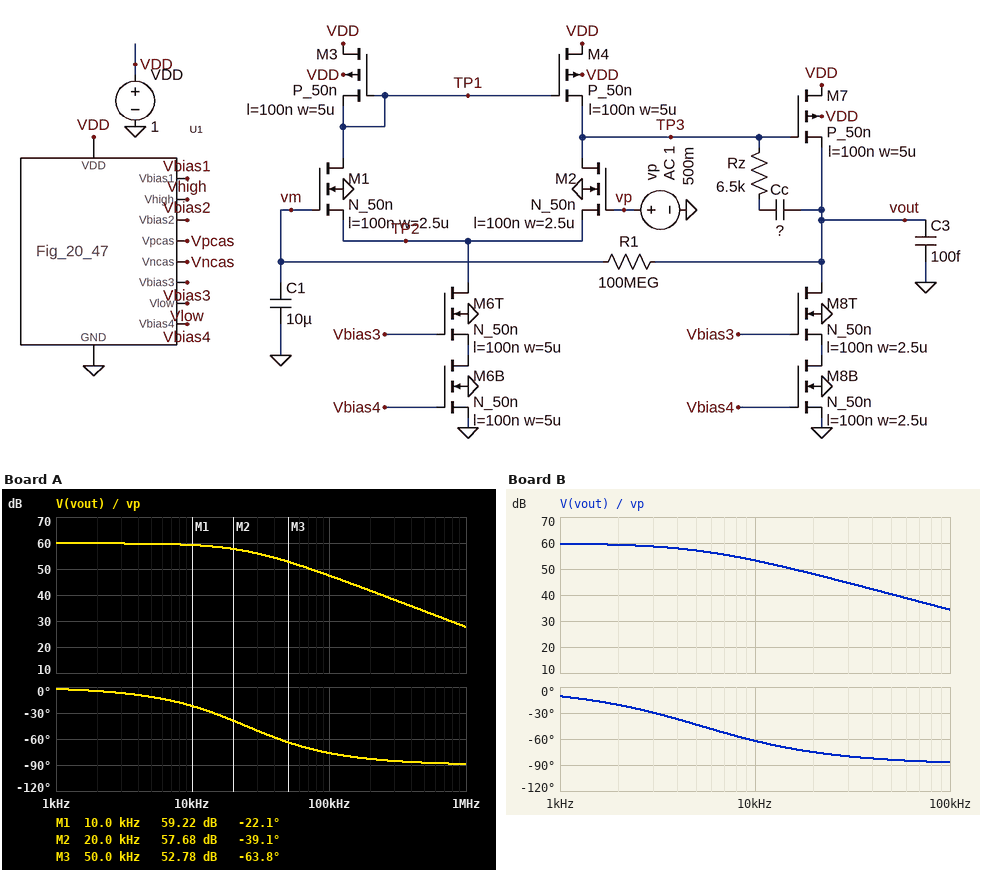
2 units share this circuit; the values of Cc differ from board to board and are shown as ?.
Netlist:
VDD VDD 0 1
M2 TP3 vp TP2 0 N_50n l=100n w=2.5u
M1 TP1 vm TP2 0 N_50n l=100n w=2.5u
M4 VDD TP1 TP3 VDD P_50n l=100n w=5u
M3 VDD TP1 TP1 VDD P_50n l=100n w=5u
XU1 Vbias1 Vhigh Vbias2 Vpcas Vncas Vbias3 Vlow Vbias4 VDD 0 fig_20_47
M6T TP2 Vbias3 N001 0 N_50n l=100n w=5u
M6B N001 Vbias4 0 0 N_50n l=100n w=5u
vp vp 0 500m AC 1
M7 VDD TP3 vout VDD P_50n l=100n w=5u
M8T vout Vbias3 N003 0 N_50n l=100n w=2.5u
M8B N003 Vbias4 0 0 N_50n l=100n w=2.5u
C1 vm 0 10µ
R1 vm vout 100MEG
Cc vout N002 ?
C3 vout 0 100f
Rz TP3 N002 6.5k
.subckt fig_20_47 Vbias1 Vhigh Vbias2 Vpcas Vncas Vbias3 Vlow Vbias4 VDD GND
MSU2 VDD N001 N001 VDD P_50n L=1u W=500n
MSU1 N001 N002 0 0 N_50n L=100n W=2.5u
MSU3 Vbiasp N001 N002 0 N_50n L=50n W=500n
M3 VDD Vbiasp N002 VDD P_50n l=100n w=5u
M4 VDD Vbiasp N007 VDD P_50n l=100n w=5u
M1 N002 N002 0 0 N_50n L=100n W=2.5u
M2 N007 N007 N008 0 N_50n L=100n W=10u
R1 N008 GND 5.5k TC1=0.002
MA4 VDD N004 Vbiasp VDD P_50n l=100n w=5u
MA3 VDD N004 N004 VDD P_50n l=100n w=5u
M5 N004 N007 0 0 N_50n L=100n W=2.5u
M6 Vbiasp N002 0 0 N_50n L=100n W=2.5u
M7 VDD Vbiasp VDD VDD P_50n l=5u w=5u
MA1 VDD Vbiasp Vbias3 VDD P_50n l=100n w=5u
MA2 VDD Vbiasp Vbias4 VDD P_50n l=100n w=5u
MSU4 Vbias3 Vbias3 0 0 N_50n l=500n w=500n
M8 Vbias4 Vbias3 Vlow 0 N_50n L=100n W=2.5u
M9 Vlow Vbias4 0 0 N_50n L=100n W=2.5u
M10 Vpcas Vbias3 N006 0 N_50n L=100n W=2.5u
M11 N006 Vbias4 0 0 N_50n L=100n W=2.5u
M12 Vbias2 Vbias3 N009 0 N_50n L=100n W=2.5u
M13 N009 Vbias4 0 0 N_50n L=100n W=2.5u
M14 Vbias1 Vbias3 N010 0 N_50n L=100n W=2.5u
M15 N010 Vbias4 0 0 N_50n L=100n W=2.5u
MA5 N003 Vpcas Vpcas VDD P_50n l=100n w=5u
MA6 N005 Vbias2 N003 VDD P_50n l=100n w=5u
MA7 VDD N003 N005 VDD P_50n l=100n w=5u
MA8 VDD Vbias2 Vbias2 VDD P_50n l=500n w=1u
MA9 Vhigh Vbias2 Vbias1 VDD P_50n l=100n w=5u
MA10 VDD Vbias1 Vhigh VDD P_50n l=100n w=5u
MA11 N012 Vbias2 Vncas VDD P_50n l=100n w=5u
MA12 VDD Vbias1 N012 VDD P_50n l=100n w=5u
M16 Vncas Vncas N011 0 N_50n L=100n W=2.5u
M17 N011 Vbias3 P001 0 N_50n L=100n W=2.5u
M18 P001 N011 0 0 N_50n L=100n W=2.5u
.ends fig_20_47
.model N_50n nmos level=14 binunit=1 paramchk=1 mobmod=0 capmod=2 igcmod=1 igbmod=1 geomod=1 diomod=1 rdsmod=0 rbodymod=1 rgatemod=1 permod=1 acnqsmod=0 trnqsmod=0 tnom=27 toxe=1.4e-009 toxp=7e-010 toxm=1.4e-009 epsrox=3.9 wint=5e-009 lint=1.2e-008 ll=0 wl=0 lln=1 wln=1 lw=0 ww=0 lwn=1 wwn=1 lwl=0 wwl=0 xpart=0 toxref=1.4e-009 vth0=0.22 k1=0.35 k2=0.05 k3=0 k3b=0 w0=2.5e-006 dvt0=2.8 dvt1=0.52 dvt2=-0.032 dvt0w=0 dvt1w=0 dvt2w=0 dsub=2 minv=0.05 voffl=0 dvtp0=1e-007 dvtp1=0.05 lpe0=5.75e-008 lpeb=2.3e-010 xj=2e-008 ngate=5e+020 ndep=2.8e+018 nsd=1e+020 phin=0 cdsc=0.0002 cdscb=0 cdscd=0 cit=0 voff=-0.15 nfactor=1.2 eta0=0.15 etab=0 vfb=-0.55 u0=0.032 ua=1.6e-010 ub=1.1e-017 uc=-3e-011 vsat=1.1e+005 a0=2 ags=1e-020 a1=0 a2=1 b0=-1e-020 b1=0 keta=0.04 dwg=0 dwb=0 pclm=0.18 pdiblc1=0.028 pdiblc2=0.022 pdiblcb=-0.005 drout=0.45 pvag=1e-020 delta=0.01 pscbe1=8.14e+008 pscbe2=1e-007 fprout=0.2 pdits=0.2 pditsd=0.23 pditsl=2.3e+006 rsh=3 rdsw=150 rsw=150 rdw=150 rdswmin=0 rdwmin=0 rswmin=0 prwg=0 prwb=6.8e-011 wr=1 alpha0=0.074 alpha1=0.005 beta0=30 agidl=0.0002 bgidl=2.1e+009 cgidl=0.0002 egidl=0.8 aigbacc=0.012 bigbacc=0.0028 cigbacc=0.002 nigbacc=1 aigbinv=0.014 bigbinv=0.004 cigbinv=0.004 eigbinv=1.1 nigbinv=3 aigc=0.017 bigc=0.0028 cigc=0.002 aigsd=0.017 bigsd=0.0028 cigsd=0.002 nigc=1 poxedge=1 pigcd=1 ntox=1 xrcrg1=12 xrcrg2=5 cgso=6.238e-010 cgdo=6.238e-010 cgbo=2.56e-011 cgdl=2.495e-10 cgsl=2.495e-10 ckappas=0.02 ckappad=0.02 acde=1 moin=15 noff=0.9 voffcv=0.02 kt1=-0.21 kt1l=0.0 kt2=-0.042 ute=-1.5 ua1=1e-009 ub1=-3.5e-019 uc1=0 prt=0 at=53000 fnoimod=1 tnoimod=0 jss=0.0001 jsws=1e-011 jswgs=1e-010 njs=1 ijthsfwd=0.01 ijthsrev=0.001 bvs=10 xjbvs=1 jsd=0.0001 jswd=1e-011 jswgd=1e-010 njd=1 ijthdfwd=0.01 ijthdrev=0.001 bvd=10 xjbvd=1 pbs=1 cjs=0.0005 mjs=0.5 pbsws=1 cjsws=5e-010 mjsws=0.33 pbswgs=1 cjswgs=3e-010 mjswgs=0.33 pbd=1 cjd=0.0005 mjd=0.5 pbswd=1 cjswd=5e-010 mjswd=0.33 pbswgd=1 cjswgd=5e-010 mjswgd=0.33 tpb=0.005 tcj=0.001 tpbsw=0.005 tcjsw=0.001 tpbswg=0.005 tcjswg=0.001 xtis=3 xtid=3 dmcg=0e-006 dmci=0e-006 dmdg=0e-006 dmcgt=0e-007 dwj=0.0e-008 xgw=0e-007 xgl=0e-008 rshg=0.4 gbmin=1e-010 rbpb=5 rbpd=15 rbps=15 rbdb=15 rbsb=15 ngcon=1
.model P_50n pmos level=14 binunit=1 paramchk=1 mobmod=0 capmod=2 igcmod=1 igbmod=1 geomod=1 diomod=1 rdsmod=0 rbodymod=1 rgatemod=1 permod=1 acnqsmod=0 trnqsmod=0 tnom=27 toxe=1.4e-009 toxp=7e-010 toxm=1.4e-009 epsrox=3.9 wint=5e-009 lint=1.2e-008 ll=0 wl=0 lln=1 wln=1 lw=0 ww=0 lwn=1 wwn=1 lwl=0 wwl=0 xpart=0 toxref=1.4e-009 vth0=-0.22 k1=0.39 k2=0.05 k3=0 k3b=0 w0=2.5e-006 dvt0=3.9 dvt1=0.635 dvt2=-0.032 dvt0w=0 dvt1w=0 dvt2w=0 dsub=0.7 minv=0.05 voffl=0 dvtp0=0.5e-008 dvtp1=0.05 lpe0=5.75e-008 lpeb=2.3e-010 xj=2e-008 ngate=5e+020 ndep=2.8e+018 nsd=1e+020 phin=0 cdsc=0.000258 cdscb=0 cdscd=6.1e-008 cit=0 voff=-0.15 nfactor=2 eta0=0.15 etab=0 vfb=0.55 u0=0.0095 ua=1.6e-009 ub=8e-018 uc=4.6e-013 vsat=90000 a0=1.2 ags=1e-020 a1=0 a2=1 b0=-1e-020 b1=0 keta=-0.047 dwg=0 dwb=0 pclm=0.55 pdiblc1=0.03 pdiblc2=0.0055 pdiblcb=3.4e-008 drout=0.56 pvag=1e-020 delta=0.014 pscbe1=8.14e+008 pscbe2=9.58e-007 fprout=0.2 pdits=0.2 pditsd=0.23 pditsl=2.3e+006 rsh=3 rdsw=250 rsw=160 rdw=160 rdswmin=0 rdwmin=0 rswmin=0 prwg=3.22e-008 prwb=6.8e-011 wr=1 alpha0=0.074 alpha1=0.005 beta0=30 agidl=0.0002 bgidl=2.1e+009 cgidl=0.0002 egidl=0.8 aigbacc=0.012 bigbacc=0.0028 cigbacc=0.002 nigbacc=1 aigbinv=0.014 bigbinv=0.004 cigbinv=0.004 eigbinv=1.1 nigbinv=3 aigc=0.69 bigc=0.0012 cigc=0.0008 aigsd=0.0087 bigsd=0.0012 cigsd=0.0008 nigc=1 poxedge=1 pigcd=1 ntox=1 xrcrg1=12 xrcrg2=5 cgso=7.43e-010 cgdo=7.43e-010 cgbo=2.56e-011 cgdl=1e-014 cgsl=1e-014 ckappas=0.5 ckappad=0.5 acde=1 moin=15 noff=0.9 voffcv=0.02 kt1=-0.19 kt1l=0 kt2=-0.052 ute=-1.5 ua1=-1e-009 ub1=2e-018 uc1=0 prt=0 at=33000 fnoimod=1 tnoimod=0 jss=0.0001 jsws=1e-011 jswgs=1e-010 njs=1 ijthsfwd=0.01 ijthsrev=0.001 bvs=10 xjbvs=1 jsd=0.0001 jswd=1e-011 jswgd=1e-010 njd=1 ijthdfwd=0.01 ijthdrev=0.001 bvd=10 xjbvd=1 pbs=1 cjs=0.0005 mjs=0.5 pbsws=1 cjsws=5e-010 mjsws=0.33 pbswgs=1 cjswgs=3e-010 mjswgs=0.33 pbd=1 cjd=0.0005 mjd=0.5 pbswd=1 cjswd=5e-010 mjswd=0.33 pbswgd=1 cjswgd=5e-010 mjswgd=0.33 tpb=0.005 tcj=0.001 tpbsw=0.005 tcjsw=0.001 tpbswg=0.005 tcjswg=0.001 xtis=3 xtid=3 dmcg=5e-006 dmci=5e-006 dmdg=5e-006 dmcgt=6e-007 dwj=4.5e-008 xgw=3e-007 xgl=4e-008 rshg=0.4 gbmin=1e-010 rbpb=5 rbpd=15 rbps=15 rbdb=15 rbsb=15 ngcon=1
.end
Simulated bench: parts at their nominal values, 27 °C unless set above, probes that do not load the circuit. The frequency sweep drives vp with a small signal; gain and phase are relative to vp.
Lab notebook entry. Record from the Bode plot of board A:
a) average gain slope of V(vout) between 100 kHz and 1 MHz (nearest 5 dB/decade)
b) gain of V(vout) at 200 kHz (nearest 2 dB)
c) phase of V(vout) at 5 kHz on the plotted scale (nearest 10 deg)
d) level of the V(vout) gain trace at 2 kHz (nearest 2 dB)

-20 dB/decade
42 dB
-10 deg
60 dB
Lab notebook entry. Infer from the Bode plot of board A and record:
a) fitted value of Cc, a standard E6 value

1 pF
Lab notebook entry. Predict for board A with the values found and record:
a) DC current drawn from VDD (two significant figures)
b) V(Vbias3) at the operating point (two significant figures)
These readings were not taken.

140 µA
540 mV
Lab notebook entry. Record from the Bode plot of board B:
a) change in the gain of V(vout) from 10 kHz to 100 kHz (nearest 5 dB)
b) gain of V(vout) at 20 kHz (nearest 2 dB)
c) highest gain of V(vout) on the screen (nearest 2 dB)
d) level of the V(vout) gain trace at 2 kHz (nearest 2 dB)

-20 dB
48 dB
60 dB
60 dB
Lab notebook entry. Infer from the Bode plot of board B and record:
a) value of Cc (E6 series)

4.7 pF
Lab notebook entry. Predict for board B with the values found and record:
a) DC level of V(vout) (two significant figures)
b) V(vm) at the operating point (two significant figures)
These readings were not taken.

520 mV
500 mV
